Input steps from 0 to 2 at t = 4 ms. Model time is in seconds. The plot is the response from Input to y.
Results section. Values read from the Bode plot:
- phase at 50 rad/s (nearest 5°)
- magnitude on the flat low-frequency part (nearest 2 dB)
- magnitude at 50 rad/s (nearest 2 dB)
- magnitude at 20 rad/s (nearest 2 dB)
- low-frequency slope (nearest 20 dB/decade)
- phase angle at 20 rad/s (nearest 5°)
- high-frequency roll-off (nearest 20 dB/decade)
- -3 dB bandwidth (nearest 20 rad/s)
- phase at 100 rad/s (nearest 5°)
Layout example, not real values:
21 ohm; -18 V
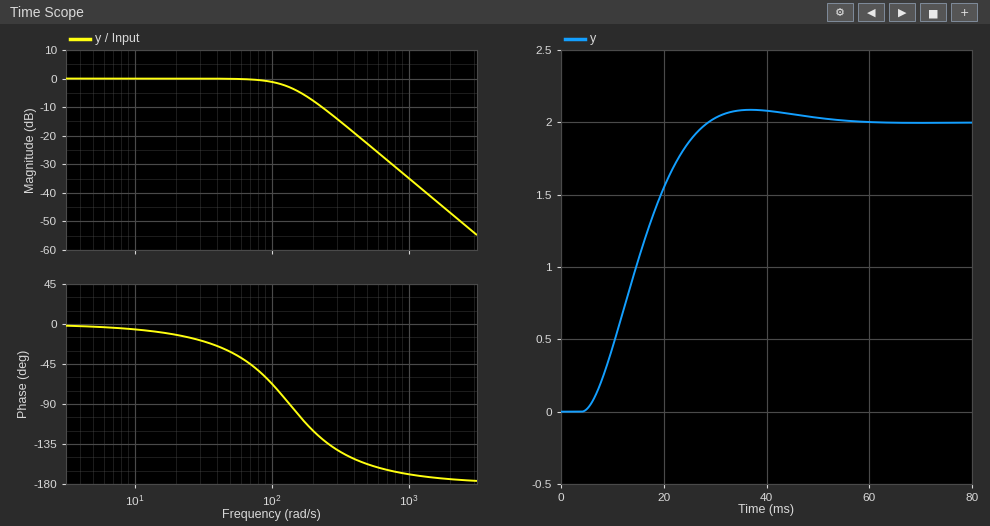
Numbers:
-30°; 0 dB; 0 dB; 0 dB; 0 dB/decade; -10°; -40 dB/decade; 140 rad/s; -65°
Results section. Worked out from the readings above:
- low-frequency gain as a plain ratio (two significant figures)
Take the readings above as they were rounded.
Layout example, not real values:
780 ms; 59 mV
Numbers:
1.0
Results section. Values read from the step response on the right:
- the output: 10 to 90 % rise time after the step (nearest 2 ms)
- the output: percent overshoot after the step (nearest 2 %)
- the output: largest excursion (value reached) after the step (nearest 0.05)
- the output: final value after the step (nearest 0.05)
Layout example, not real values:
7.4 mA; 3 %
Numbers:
16 ms; 4 %; 2.10; 2.00
